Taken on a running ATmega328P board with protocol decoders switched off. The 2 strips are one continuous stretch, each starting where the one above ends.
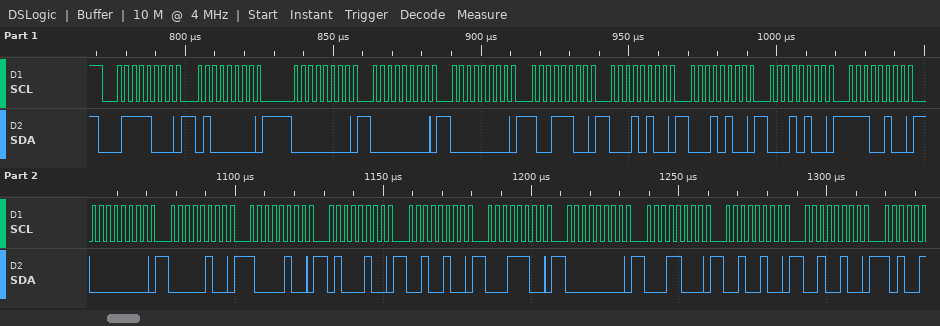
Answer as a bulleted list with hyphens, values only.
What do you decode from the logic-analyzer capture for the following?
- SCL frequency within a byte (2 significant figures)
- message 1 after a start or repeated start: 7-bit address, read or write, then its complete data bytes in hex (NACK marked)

- 400 kHz
- 0x3C write: 40 00 00 00 9C 14 14 14 E4 00 04 84 44 24 1C 00 18 24 24
